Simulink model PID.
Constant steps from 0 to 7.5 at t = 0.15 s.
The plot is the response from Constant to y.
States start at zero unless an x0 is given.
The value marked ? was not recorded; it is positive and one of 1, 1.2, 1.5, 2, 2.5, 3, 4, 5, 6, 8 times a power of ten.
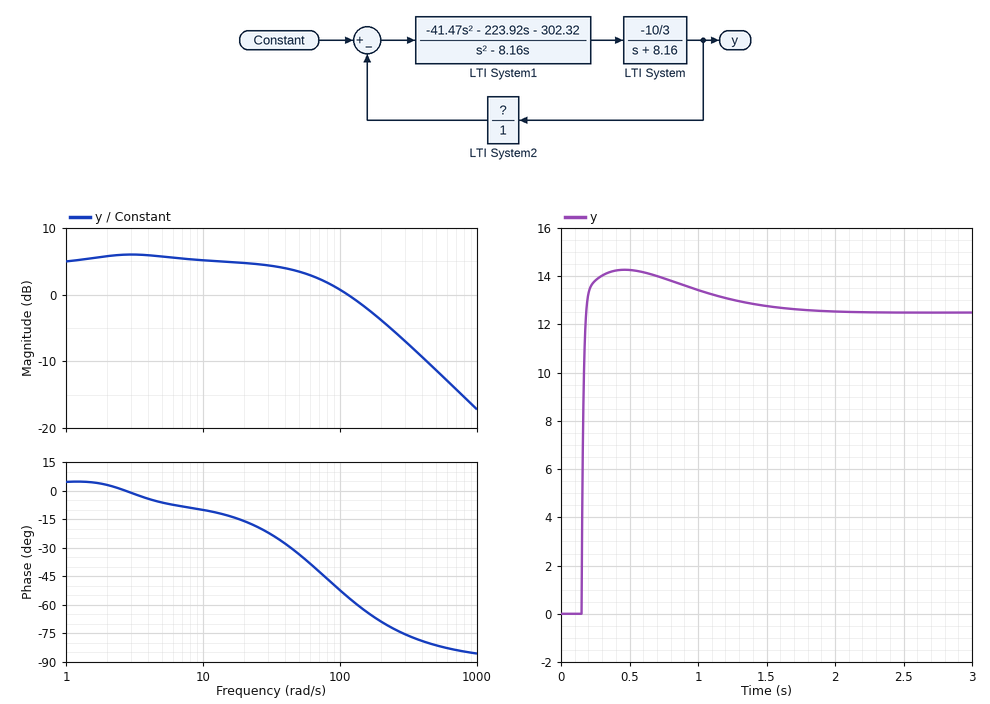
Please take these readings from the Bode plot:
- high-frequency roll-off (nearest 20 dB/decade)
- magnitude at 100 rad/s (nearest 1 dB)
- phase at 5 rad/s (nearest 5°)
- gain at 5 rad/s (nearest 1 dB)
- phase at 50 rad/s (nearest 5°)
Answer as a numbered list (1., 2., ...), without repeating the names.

1. -20 dB/decade
2. 1 dB
3. -5°
4. 6 dB
5. -35°
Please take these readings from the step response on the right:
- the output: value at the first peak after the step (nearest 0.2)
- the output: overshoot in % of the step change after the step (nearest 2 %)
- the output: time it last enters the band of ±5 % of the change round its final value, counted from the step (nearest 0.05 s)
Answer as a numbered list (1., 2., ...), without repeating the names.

1. 14.2
2. 14 %
3. 1.05 s
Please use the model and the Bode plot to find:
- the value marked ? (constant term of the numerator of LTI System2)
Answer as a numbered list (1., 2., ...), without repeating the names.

1. 0.6
